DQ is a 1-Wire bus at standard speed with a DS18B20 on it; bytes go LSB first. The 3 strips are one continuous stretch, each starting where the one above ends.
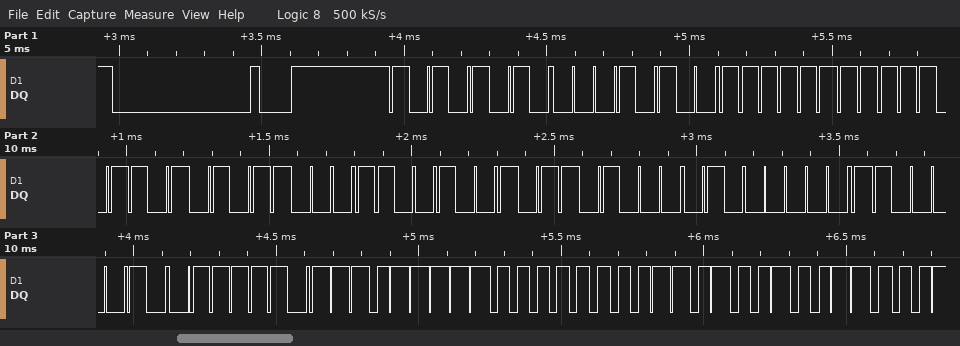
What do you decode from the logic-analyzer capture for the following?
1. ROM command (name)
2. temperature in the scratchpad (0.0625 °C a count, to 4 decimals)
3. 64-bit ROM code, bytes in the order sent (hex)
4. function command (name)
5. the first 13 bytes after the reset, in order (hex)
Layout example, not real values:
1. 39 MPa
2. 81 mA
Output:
1. Match ROM
2. 15.6875 °C
3. 28 FF B7 1A 93 16 02 43
4. Read Scratchpad
5. 55 28 FF B7 1A 93 16 02 43 BE FB 00 4B
